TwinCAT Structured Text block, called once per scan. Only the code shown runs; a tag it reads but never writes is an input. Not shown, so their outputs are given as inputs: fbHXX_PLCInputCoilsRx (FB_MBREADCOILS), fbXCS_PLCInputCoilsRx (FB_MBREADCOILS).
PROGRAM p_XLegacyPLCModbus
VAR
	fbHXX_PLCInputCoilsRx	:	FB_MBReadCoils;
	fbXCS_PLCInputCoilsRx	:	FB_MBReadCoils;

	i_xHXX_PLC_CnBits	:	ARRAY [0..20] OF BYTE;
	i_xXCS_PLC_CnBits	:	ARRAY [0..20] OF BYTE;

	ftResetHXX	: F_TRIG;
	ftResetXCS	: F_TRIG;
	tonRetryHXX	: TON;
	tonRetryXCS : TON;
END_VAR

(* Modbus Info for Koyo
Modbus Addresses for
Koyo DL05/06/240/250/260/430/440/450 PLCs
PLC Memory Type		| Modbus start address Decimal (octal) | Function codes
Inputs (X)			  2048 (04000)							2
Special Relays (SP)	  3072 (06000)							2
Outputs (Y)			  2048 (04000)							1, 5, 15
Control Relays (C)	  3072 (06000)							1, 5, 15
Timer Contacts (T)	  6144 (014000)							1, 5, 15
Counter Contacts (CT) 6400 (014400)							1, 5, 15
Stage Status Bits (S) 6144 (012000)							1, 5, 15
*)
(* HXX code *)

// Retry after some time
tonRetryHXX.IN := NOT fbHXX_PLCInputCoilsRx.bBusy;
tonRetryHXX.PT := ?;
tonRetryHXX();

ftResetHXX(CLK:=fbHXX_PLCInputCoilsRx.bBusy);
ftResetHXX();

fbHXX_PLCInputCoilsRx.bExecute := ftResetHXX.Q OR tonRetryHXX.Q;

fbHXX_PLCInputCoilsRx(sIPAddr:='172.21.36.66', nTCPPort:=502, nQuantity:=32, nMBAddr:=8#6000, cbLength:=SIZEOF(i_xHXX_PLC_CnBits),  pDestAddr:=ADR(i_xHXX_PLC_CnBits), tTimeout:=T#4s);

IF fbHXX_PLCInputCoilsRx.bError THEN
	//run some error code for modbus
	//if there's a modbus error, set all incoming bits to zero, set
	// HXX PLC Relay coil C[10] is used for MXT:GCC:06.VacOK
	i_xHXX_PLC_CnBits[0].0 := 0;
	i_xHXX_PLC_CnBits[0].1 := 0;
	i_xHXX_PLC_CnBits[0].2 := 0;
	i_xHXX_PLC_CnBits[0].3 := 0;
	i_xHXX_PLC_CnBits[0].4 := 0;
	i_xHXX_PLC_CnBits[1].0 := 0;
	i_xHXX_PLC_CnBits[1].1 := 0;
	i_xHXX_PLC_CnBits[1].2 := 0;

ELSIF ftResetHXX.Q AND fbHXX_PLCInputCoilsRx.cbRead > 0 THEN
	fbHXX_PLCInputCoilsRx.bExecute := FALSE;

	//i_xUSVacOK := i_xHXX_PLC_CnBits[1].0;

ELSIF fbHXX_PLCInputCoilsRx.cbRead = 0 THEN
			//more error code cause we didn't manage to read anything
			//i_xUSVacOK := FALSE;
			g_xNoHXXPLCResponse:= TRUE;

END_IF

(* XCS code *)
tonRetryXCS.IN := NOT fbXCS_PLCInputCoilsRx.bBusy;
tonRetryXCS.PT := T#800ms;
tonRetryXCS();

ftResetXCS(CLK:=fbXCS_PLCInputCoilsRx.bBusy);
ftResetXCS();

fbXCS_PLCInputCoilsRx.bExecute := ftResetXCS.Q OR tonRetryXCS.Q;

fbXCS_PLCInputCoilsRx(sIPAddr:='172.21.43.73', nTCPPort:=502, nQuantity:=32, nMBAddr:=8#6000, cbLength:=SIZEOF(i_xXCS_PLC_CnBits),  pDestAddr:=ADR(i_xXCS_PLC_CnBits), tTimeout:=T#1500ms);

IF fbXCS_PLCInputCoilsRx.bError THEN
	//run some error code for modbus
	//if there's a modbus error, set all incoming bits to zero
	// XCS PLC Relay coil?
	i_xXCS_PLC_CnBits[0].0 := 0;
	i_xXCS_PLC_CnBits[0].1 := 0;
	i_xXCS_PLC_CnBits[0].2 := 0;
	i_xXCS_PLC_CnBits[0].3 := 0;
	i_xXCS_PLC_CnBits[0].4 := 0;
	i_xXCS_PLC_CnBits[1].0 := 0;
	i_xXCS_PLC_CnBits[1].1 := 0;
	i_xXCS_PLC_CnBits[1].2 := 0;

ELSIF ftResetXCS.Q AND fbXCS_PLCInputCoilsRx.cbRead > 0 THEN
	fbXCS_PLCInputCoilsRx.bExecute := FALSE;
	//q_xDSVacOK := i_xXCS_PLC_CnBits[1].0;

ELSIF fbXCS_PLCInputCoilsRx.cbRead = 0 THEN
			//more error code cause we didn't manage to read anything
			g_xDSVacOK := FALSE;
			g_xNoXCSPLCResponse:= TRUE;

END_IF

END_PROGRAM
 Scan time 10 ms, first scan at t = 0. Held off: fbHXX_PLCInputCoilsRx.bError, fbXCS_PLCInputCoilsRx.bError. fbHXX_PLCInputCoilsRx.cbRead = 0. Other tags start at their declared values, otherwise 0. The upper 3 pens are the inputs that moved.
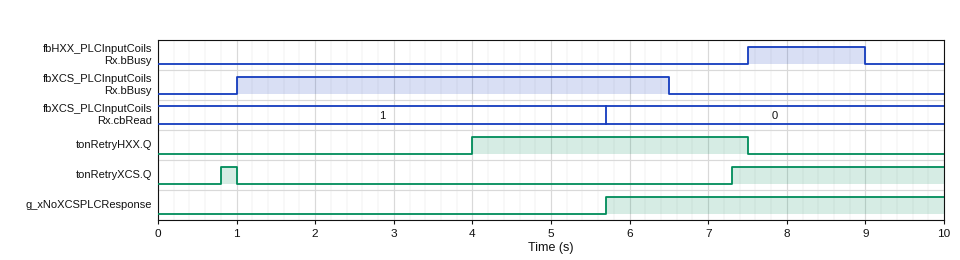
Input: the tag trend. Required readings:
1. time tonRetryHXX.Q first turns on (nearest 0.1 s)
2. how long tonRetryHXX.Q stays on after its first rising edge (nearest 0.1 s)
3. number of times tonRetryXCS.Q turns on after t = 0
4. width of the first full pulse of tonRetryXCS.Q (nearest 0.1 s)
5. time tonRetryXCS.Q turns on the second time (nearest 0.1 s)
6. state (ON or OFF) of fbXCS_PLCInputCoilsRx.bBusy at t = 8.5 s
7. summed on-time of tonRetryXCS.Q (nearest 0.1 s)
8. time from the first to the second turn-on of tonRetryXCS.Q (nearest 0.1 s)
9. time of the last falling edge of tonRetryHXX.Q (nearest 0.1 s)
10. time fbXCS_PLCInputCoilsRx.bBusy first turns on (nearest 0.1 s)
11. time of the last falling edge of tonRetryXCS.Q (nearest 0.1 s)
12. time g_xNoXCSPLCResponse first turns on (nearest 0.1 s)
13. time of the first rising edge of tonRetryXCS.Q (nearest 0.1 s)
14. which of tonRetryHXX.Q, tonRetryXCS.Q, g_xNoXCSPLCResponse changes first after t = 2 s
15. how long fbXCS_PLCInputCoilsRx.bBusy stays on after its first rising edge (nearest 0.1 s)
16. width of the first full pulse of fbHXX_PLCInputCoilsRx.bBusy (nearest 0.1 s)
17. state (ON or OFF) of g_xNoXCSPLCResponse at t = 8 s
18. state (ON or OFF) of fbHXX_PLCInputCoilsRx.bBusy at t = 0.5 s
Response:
4.0 s
3.5 s
2
0.2 s
7.3 s
OFF
2.9 s
6.5 s
7.5 s
1.0 s
1.0 s
5.7 s
0.8 s
tonRetryHXX.Q
5.5 s
1.5 s
ON
OFF
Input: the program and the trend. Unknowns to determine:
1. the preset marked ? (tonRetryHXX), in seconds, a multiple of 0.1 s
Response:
4.0 s
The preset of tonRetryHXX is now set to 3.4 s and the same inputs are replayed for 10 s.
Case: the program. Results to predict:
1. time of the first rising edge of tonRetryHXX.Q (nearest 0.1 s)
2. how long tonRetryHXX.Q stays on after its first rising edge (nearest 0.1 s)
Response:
3.4 s
4.1 s
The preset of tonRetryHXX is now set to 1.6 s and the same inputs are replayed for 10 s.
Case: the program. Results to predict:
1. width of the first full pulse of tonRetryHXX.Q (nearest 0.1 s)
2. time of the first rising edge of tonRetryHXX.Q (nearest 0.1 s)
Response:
5.9 s
1.6 s
